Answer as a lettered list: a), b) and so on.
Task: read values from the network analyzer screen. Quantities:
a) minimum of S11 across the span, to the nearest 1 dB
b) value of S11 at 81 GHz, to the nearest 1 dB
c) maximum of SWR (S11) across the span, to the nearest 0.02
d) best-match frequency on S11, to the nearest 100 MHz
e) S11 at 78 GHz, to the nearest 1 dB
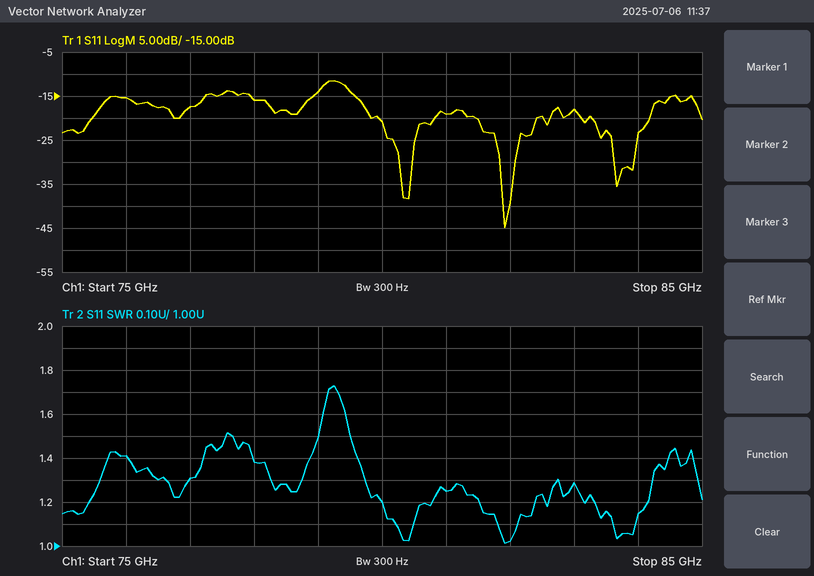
a) -45 dB
b) -19 dB
c) 1.72
d) 81.9 GHz
e) -16 dB
